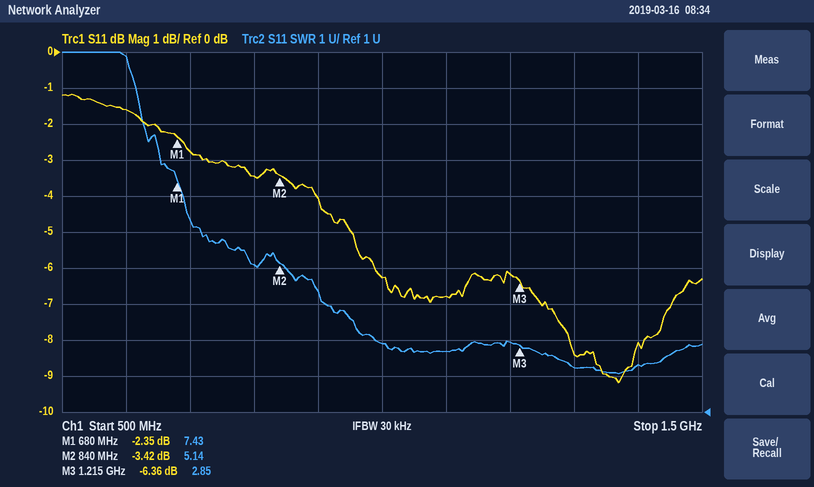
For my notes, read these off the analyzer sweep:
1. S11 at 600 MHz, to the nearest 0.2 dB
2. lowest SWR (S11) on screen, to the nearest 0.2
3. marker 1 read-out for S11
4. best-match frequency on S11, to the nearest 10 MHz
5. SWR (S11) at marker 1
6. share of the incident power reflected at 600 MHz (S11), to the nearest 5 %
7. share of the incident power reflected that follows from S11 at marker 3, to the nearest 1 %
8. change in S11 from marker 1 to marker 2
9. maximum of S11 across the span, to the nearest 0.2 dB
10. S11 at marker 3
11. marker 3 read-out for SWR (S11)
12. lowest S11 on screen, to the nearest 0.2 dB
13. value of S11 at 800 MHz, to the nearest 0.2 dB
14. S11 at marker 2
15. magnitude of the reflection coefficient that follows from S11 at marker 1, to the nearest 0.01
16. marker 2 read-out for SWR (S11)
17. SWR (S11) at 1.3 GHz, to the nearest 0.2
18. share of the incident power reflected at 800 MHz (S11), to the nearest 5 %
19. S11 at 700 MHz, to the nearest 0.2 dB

-1.6 dB
2.0
-2.35 dB
1.37 GHz
7.43
70 %
23 %
-1.07 dB
-1.2 dB
-6.36 dB
2.85
-9.2 dB
-3.4 dB
-3.42 dB
0.76
5.14
2.2
45 %
-2.8 dB
